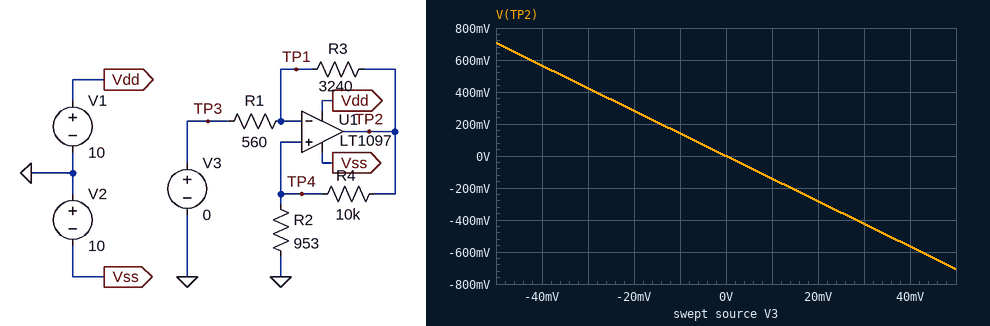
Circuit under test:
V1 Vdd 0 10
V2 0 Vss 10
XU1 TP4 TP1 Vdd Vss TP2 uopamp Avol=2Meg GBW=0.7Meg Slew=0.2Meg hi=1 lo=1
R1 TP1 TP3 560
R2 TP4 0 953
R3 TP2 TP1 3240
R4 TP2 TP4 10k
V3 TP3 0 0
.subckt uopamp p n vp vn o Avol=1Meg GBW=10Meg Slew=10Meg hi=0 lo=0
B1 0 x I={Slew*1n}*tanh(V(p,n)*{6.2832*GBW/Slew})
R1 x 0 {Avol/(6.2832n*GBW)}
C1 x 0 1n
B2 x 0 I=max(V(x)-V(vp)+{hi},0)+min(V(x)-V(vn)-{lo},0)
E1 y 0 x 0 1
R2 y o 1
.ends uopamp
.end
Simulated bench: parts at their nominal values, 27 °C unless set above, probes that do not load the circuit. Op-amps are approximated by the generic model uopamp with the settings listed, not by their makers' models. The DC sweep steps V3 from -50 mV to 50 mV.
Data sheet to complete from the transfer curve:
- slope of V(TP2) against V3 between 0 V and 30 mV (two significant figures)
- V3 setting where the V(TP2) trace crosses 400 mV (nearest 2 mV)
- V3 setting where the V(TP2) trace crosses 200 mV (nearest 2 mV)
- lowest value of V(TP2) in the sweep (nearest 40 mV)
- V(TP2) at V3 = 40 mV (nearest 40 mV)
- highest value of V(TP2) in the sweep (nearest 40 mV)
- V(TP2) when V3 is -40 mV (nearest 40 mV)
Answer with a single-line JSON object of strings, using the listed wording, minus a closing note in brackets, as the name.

{"slope of V(TP2) against V3 between 0 V and 30 mV": "-14 V/V", "V3 setting where the V(TP2) trace crosses 400 mV": "-28 mV", "V3 setting where the V(TP2) trace crosses 200 mV": "-14 mV", "lowest value of V(TP2) in the sweep": "-720 mV", "V(TP2) at V3 = 40 mV": "-560 mV", "highest value of V(TP2) in the sweep": "720 mV", "V(TP2) when V3 is -40 mV": "560 mV"}
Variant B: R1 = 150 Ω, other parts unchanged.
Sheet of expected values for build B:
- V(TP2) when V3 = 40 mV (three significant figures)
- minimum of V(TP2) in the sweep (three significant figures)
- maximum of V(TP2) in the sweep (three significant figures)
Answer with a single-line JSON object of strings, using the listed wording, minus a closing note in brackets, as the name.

{"V(TP2) when V3 = 40 mV": "894 mV", "minimum of V(TP2) in the sweep": "-1.12 V", "maximum of V(TP2) in the sweep": "1.12 V"}
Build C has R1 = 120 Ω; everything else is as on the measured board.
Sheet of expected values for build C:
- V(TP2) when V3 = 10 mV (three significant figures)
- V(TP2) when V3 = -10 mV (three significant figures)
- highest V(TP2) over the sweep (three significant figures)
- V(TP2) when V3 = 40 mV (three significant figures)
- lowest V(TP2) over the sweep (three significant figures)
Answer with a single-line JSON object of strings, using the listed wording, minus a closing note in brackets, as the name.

{"V(TP2) when V3 = 10 mV": "188 mV", "V(TP2) when V3 = -10 mV": "-188 mV", "highest V(TP2) over the sweep": "940 mV", "V(TP2) when V3 = 40 mV": "752 mV", "lowest V(TP2) over the sweep": "-940 mV"}
